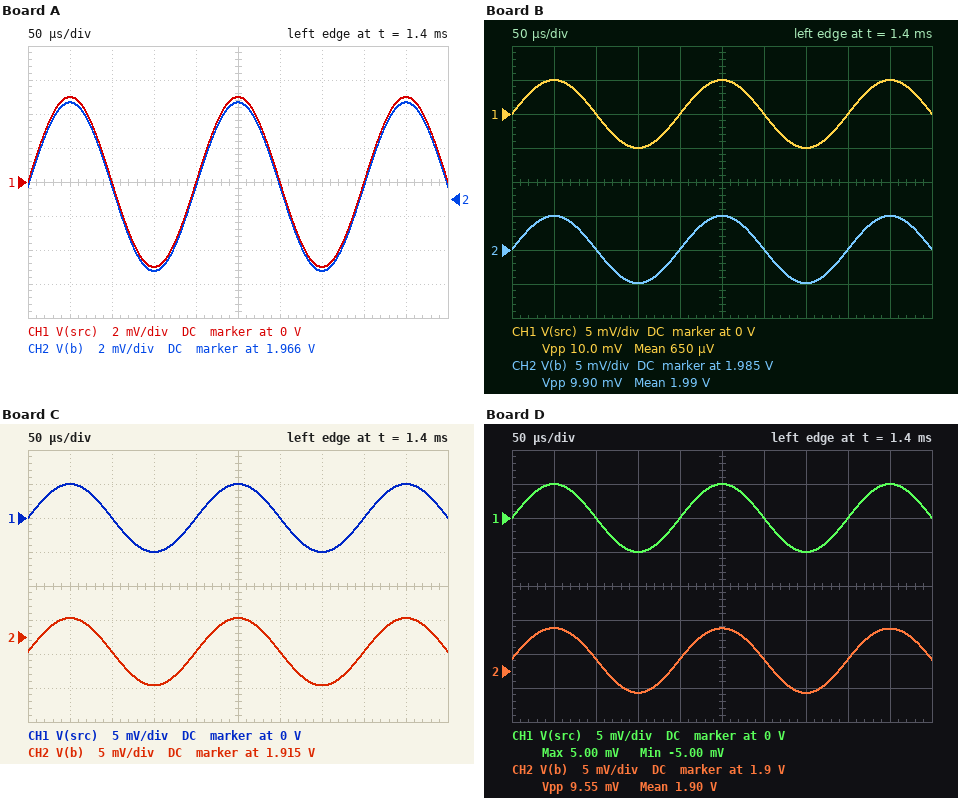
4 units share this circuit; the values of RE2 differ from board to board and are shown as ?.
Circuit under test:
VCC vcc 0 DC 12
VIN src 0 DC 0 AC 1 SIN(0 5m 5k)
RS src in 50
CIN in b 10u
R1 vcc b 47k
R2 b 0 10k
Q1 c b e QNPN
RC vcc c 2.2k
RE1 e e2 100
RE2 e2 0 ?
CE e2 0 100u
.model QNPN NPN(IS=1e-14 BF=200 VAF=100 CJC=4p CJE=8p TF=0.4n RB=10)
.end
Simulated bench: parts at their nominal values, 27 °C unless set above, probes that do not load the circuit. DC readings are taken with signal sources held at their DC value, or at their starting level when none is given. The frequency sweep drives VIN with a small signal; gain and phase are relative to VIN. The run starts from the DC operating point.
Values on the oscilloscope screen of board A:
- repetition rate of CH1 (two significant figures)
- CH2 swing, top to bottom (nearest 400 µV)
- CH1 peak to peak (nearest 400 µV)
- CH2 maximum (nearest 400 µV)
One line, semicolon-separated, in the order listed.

5.0 kHz; 10.0 mV; 10.0 mV; 1.9716 V
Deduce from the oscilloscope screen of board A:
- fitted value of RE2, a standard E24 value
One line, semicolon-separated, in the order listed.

270 Ω
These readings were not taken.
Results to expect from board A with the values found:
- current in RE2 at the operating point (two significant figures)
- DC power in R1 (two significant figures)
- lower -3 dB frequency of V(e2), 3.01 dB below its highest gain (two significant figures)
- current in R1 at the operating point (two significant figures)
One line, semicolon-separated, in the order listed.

3.5 mA; 2.1 mW; 1.8 Hz; 210 µA
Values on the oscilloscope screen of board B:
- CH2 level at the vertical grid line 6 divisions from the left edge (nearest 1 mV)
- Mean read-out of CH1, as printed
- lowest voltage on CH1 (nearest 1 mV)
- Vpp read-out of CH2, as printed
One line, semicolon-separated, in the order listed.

1.985 V; 650 µV; -5 mV; 9.90 mV
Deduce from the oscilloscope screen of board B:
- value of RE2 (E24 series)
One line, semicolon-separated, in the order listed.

330 Ω
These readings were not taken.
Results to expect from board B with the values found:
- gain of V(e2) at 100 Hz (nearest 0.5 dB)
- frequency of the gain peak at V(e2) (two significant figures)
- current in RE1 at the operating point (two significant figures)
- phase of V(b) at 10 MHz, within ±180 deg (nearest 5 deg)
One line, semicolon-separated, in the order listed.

-17.0 dB; 6.4 Hz; 3.0 mA; -10 deg
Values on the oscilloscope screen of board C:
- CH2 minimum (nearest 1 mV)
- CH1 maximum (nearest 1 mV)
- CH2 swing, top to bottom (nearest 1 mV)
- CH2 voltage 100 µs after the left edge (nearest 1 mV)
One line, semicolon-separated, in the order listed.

1.908 V; 5 mV; 10 mV; 1.913 V
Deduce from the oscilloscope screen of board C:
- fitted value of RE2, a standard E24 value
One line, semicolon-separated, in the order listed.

160 Ω
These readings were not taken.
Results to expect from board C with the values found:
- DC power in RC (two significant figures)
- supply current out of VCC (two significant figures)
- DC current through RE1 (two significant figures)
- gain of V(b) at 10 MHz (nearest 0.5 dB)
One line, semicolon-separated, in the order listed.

48 mW; 4.9 mA; 4.7 mA; -1.5 dB
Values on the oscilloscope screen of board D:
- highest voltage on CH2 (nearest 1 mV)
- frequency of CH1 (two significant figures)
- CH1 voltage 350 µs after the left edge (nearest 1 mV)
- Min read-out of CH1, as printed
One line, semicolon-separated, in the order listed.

1.906 V; 5.0 kHz; -5 mV; -5.00 mV
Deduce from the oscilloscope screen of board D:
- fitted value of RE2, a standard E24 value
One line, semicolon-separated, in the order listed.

150 Ω
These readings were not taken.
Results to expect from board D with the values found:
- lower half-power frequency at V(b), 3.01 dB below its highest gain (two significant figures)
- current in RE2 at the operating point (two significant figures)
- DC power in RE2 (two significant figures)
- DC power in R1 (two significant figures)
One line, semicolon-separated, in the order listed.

6.4 Hz; 4.8 mA; 3.5 mW; 2.2 mW
